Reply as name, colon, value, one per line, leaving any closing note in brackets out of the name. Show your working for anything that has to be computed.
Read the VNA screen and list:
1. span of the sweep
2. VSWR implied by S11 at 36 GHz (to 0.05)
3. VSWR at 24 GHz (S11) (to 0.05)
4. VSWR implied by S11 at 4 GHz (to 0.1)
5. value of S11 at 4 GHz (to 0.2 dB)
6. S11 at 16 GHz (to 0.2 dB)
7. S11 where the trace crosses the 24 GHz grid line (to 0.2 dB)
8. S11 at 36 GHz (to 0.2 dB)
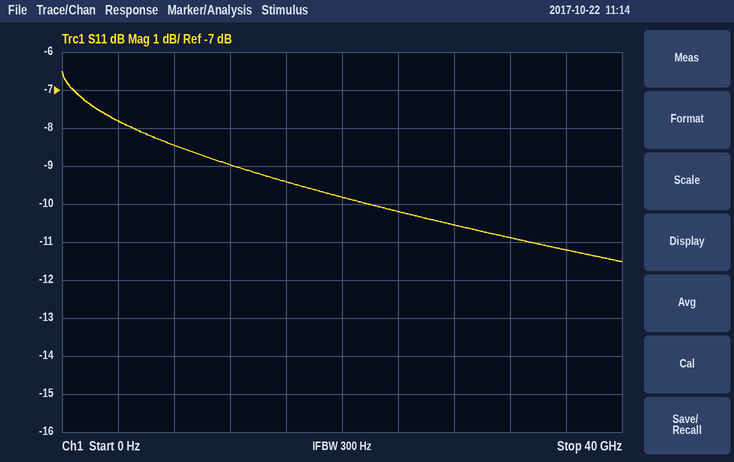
span of the sweep: 40 GHz
VSWR implied by S11 at 36 GHz: |Γ| = 10^(-11.2/20) = 0.2754; VSWR = (1 + 0.2754)/(1 − 0.2754) ≈ 1.76, so 1.75 to the nearest 0.05
VSWR at 24 GHz (S11): |Γ| = 10^(-10.2/20) = 0.3090; VSWR = (1 + 0.3090)/(1 − 0.3090) ≈ 1.89, so 1.90 to the nearest 0.05
VSWR implied by S11 at 4 GHz: |Γ| = 10^(-7.8/20) = 0.4074; VSWR = (1 + 0.4074)/(1 − 0.4074) ≈ 2.4
value of S11 at 4 GHz: -7.8 dB
S11 at 16 GHz: -9.4 dB
S11 where the trace crosses the 24 GHz grid line: -10.2 dB
S11 at 36 GHz: -11.2 dB
